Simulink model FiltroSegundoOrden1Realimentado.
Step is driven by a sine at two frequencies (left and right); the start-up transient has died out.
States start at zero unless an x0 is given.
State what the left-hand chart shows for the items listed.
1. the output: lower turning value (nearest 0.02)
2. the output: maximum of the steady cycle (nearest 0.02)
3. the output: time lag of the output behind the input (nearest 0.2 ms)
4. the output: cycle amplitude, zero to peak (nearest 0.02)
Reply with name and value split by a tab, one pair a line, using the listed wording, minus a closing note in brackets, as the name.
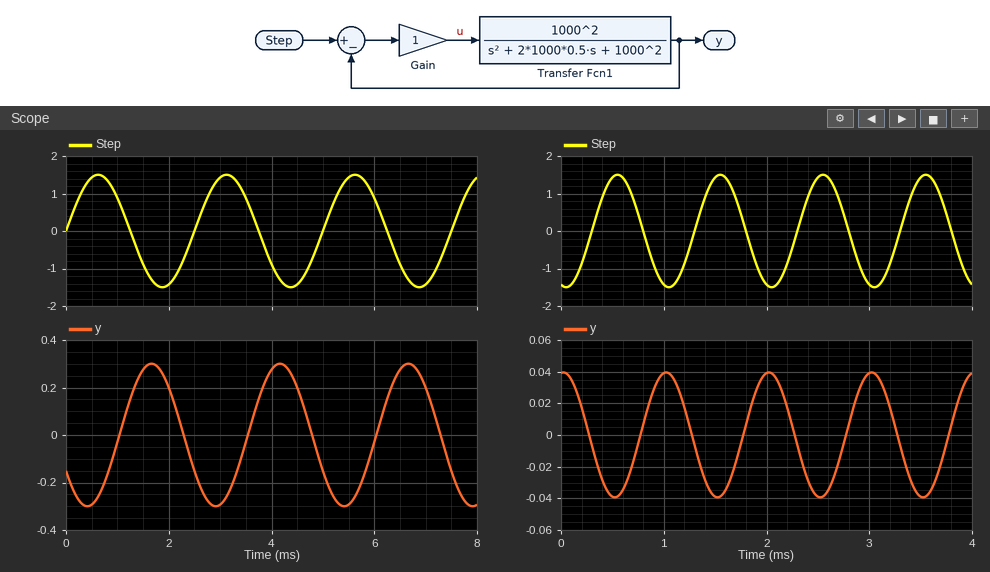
the output: lower turning value	-0.30
the output: maximum of the steady cycle	0.30
the output: time lag of the output behind the input	1.0 ms
the output: cycle amplitude, zero to peak	0.30
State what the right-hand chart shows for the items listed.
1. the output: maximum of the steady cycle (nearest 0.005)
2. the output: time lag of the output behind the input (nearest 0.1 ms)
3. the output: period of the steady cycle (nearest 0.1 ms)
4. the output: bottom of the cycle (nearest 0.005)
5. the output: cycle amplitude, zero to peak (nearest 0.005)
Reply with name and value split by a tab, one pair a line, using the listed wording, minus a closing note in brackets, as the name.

the output: maximum of the steady cycle	0.040
the output: time lag of the output behind the input	0.5 ms
the output: period of the steady cycle	1.0 ms
the output: bottom of the cycle	-0.040
the output: cycle amplitude, zero to peak	0.040
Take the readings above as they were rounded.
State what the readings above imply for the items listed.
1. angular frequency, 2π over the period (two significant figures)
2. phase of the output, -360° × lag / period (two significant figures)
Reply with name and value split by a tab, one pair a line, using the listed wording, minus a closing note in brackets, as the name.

angular frequency, 2π over the period	6.3 rad/ms
phase of the output, -360° × lag / period	-180°
